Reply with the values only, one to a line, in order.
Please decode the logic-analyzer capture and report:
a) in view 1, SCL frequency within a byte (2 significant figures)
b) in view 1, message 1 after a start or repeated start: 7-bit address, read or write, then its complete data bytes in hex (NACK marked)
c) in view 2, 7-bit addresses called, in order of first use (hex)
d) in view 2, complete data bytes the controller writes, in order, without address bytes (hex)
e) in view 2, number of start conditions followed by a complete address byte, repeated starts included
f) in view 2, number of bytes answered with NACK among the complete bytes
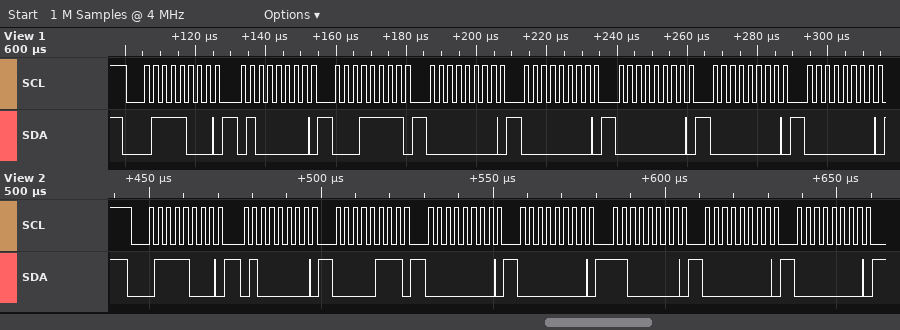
400 kHz
0x3C write: 40 1F 00 00 00 00 00
0x3C
40 07 00 00 C0 00 00
1
0
